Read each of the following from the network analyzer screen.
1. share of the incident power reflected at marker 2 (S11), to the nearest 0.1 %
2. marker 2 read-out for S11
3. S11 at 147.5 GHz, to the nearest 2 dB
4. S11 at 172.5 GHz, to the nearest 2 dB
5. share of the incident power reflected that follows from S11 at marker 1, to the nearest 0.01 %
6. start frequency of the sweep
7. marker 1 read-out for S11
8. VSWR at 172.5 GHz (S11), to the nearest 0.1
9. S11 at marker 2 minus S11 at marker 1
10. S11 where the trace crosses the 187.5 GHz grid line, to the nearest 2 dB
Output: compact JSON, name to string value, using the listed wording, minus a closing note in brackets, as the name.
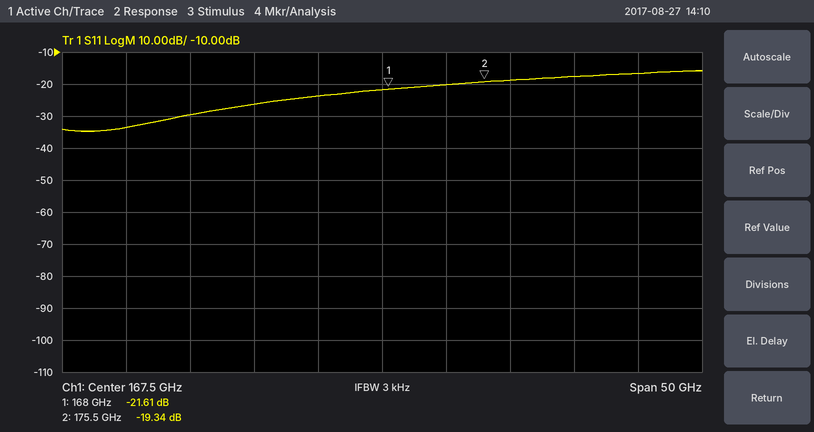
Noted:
{"share of the incident power reflected at marker 2 (S11), to the nearest 0.1 %": "1.2 %", "marker 2 read-out for S11": "-19.34 dB", "S11 at 147.5 GHz, to the nearest 2 dB": "-34 dB", "S11 at 172.5 GHz, to the nearest 2 dB": "-20 dB", "share of the incident power reflected that follows from S11 at marker 1, to the nearest 0.01 %": "0.69 %", "start frequency of the sweep": "142.5 GHz", "marker 1 read-out for S11": "-21.61 dB", "VSWR at 172.5 GHz (S11), to the nearest 0.1": "1.2", "S11 at marker 2 minus S11 at marker 1": "2.27 dB", "S11 where the trace crosses the 187.5 GHz grid line, to the nearest 2 dB": "-16 dB"}
